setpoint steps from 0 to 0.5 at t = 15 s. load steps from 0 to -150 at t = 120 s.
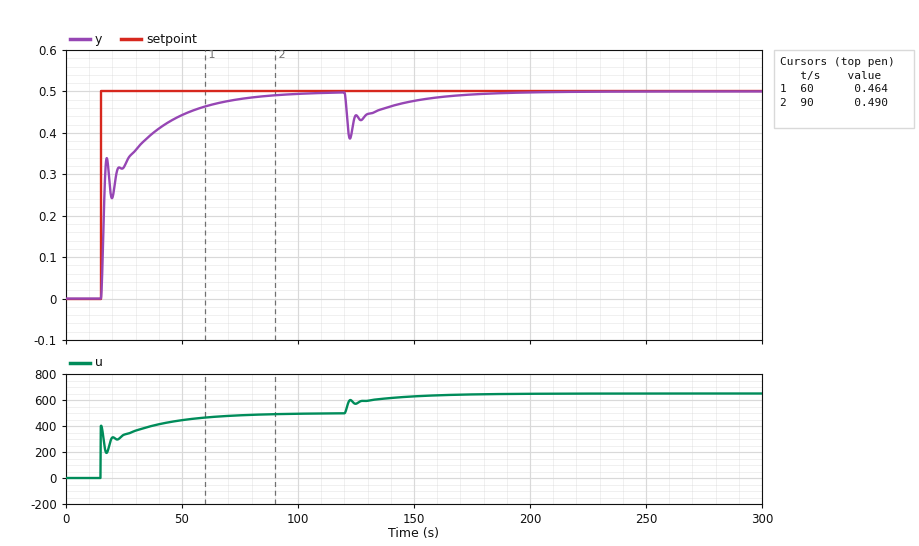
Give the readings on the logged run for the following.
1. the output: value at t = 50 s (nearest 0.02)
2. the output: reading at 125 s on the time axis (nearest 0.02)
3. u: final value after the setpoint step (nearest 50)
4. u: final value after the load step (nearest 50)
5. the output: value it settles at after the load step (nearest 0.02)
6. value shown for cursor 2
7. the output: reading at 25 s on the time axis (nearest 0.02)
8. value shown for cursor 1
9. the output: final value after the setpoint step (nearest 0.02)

0.44
0.44
500
650
0.50
0.490
0.32
0.464
0.50
